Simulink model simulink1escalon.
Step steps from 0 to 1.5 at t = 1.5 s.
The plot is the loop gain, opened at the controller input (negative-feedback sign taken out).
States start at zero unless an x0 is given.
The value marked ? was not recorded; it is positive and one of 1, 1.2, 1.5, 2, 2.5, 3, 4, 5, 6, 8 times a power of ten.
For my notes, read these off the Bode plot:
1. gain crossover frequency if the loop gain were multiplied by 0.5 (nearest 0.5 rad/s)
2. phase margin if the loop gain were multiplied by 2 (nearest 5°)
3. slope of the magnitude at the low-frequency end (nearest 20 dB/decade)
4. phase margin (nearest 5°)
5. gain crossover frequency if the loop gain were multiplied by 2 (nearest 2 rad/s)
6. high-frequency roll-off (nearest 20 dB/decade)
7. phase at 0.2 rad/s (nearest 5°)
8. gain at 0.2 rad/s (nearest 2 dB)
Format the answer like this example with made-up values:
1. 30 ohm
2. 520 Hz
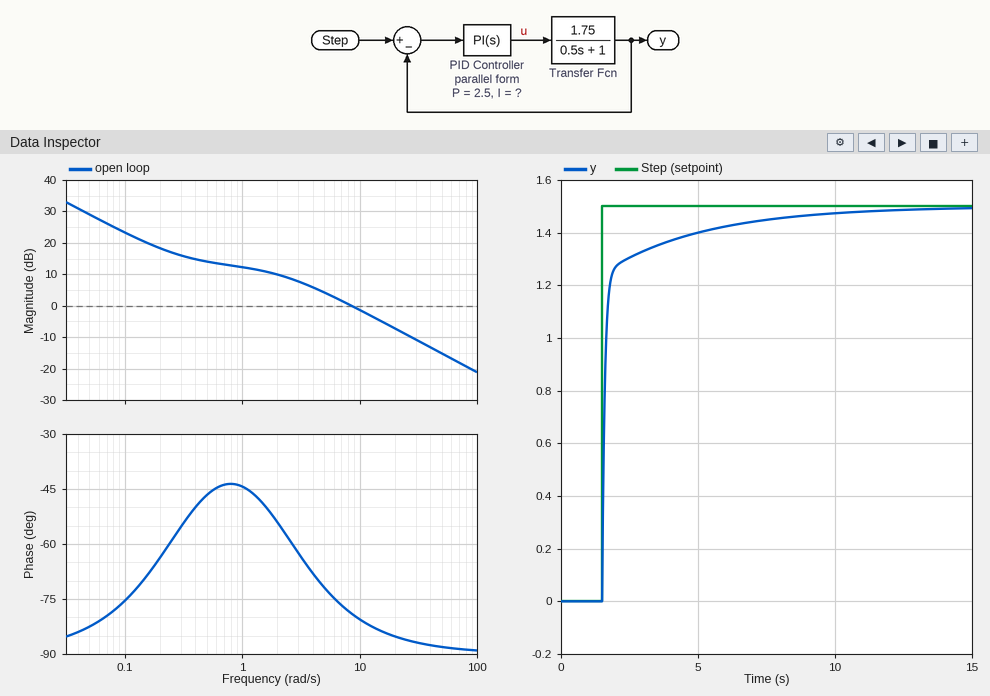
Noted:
1. 4.0 rad/s
2. 95°
3. -20 dB/decade
4. 100°
5. 18 rad/s
6. -20 dB/decade
7. -65°
8. 18 dB
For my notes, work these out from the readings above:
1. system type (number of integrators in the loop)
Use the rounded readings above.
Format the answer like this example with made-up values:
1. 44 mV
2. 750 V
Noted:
1. 1
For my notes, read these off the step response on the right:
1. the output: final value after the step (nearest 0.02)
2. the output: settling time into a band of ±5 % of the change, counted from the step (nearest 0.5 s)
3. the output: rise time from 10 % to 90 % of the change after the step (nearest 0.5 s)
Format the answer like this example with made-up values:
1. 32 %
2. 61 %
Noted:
1. 1.50
2. 4.5 s
3. 2.0 s
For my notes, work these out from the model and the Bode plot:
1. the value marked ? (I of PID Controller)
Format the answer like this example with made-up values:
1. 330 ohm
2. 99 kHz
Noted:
1. 0.8
